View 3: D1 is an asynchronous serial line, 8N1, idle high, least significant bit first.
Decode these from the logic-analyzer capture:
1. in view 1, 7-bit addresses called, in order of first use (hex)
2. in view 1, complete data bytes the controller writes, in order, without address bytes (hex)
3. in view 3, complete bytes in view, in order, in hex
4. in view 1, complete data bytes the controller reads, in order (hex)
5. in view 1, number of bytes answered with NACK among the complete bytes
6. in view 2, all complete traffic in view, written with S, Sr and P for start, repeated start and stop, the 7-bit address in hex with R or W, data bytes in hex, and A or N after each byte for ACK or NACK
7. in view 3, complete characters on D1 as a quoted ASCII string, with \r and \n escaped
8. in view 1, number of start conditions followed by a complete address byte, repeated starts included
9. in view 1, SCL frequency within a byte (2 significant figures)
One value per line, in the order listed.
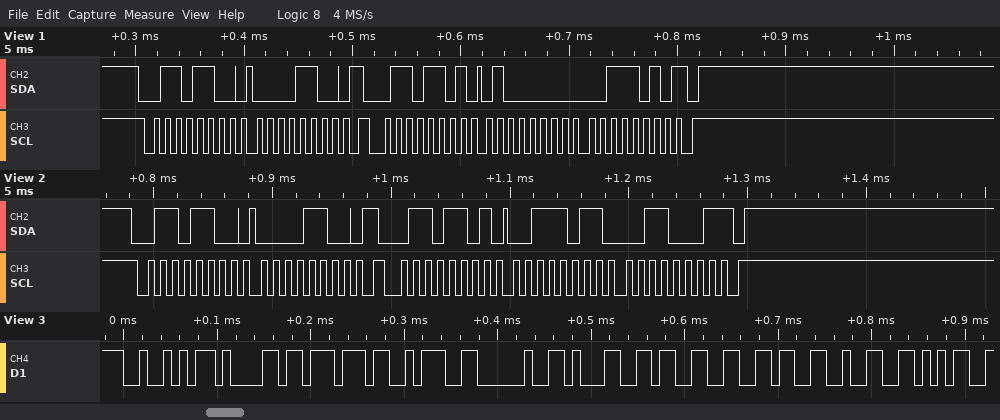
0x36
0C
0x52 0x61 0x77 0x3A 0x20 0x31 0x33 0x36 0x32 0x35
40 3A
1
S 36W A 0C A Sr 36R A 3B A 31 N P
"Raw: 13625"
2
100 kHz
